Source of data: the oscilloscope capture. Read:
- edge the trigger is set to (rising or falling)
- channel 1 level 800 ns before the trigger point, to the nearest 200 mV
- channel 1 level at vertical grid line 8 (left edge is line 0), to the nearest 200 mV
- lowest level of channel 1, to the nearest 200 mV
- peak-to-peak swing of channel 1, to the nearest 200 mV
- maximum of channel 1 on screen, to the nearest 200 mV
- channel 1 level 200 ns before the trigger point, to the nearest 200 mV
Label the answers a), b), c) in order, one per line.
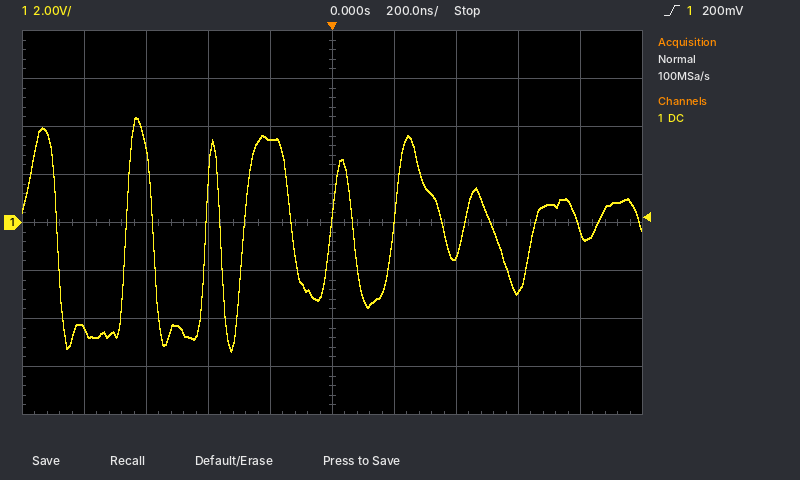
a) rising
b) -4.4 V
c) -2.8 V
d) -5.4 V
e) 9.8 V
f) 4.4 V
g) 3.4 V
